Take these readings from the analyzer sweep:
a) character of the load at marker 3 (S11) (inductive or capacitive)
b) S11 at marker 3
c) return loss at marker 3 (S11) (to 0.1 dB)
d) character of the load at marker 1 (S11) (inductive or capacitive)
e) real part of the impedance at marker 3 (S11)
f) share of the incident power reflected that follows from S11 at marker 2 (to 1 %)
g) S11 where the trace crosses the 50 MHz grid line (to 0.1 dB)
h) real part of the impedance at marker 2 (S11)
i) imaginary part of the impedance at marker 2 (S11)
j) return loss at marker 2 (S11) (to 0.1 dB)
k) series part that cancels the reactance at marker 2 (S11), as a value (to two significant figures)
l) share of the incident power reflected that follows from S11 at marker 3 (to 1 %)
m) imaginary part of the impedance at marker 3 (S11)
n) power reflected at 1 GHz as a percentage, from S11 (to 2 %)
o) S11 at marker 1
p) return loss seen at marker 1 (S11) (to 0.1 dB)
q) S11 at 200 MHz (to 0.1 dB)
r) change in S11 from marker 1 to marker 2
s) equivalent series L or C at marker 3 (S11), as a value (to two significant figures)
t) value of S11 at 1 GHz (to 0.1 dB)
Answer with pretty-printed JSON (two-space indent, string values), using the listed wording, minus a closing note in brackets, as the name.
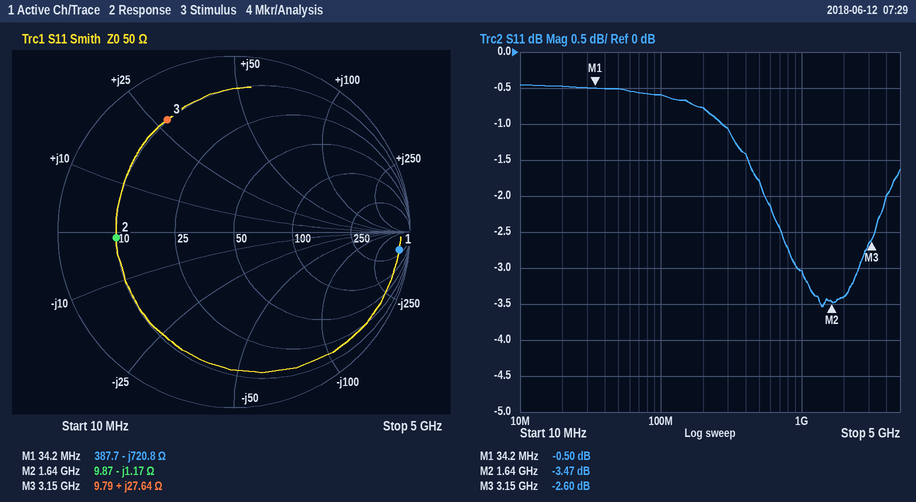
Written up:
{
  "character of the load at marker 3 (S11)": "inductive",
  "S11 at marker 3": "-2.60 dB",
  "return loss at marker 3 (S11)": "2.6 dB",
  "character of the load at marker 1 (S11)": "capacitive",
  "real part of the impedance at marker 3": "9.79 Ω",
  "share of the incident power reflected that follows from S11 at marker 2": "45 %",
  "S11 where the trace crosses the 50 MHz grid line": "-0.5 dB",
  "real part of the impedance at marker 2": "9.87 Ω",
  "imaginary part of the impedance at marker 2": "-1.17 Ω",
  "return loss at marker 2 (S11)": "3.5 dB",
  "series part that cancels the reactance at marker 2 (S11), as a value": "110 pH",
  "share of the incident power reflected that follows from S11 at marker 3": "55 %",
  "imaginary part of the impedance at marker 3": "+27.64 Ω",
  "power reflected at 1 GHz as a percentage, from S11": "50 %",
  "S11 at marker 1": "-0.50 dB",
  "return loss seen at marker 1 (S11)": "0.5 dB",
  "S11 at 200 MHz": "-0.8 dB",
  "change in S11 from marker 1 to marker 2": "-2.97 dB",
  "equivalent series L or C at marker 3 (S11), as a value": "1.4 nH",
  "value of S11 at 1 GHz": "-3.0 dB"
}
